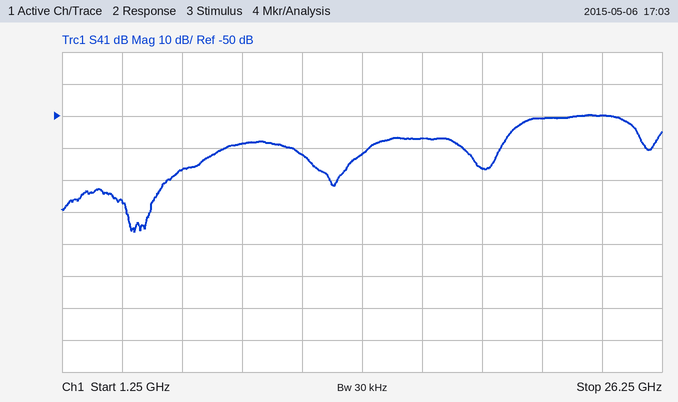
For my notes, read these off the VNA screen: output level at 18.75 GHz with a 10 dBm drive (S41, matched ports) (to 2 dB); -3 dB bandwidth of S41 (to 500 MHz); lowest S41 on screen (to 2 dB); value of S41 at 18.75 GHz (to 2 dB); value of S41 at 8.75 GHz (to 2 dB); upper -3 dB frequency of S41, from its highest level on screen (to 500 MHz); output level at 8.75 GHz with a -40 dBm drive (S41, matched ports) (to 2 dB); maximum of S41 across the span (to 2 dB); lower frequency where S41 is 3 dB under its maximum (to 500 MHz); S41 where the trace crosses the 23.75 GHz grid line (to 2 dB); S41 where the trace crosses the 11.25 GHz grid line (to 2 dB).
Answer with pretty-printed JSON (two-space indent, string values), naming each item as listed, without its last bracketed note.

{
  "output level at 18.75 GHz with a 10 dBm drive (S41, matched ports)": "-56 dBm",
  "-3 dB bandwidth of S41": "4.5 GHz",
  "lowest S41 on screen": "-86 dB",
  "value of S41 at 18.75 GHz": "-66 dB",
  "value of S41 at 8.75 GHz": "-58 dB",
  "upper -3 dB frequency of S41, from its highest level on screen": "25.0 GHz",
  "output level at 8.75 GHz with a -40 dBm drive (S41, matched ports)": "-98 dBm",
  "maximum of S41 across the span": "-50 dB",
  "lower frequency where S41 is 3 dB under its maximum": "20.5 GHz",
  "S41 where the trace crosses the 23.75 GHz grid line": "-50 dB",
  "S41 where the trace crosses the 11.25 GHz grid line": "-62 dB"
}
